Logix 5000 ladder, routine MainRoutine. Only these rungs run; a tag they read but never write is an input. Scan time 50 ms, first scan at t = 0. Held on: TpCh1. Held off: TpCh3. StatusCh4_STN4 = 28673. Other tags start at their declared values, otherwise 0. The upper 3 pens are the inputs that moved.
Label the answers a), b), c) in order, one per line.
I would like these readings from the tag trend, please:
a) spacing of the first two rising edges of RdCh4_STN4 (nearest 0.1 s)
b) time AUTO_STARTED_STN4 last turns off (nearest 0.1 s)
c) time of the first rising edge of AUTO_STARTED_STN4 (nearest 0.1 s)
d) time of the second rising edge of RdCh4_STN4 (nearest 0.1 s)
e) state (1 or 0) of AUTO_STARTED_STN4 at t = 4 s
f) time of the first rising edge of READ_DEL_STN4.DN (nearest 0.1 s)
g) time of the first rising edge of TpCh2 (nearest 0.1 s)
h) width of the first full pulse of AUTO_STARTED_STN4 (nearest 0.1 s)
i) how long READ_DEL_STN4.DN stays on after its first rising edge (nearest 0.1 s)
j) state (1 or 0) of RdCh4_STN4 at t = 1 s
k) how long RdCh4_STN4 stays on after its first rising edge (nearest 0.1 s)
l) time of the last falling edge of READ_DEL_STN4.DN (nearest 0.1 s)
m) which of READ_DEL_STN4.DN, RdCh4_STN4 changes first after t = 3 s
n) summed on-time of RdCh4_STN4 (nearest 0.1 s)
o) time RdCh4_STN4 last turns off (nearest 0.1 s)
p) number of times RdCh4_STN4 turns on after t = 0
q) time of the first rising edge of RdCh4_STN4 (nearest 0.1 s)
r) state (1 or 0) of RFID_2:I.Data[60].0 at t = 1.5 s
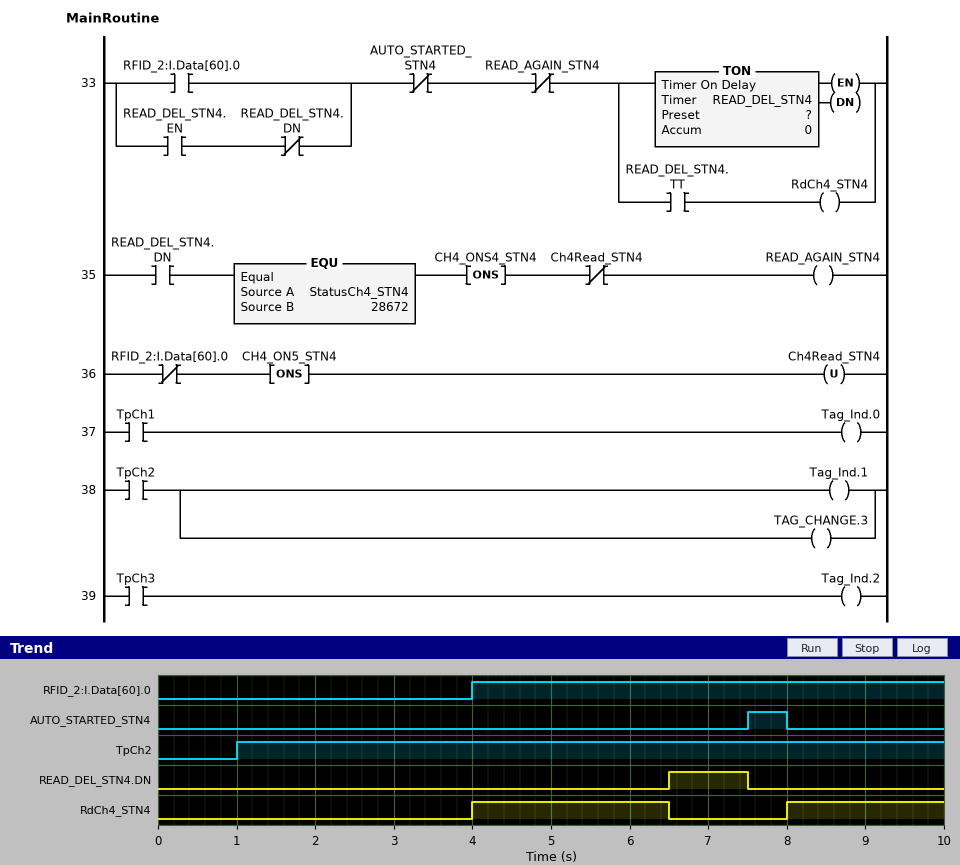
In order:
a) 4.0 s
b) 8.0 s
c) 7.5 s
d) 8.0 s
e) 0
f) 6.5 s
g) 1.0 s
h) 0.5 s
i) 1.0 s
j) 0
k) 2.5 s
l) 7.5 s
m) RdCh4_STN4
n) 4.5 s
o) 6.5 s
p) 2
q) 4.0 s
r) 0
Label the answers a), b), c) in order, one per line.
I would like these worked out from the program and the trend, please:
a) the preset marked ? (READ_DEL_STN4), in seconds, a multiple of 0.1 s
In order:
a) 2.5 s
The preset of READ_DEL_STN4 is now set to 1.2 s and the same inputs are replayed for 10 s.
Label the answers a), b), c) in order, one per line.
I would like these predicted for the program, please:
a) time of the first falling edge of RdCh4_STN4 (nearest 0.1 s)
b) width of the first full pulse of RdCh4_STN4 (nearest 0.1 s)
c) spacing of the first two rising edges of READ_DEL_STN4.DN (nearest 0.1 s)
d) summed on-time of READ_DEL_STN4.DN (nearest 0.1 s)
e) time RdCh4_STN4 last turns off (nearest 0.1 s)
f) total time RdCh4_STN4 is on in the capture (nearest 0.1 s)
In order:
a) 5.2 s
b) 1.2 s
c) 4.0 s
d) 3.1 s
e) 9.2 s
f) 2.4 s
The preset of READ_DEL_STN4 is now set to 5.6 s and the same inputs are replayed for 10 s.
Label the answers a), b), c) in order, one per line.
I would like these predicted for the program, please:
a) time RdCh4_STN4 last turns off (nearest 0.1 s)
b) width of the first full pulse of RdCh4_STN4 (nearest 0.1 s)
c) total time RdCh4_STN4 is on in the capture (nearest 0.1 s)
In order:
a) 7.5 s
b) 3.5 s
c) 5.5 s
